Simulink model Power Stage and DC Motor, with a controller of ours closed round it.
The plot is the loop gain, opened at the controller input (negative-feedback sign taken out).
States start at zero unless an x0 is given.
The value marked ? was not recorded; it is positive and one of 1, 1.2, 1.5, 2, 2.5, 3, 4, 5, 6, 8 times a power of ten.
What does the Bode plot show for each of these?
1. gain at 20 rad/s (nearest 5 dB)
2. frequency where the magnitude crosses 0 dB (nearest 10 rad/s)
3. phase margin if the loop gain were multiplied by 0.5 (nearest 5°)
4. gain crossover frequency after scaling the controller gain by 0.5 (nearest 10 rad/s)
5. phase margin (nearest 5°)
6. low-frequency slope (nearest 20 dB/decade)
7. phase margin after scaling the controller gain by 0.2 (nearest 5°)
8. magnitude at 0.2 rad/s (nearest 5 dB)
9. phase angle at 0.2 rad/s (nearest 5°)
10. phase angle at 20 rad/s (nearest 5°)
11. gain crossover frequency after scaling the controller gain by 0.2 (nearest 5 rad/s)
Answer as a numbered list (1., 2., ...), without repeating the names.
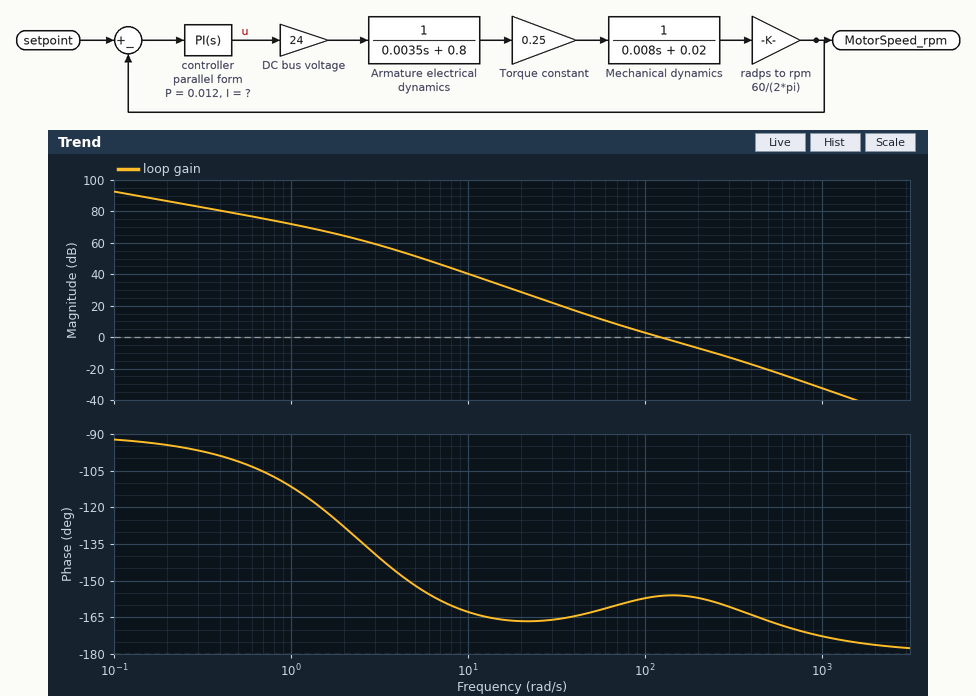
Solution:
1. 30 dB
2. 120 rad/s
3. 20°
4. 80 rad/s
5. 25°
6. -20 dB/decade
7. 15°
8. 85 dB
9. -95°
10. -165°
11. 50 rad/s
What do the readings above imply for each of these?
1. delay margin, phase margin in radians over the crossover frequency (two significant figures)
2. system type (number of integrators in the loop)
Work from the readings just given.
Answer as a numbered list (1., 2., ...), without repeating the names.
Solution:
1. 0.0036 s
2. 1
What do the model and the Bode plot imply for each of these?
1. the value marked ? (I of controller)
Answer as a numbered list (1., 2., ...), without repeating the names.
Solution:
1. 1.2
